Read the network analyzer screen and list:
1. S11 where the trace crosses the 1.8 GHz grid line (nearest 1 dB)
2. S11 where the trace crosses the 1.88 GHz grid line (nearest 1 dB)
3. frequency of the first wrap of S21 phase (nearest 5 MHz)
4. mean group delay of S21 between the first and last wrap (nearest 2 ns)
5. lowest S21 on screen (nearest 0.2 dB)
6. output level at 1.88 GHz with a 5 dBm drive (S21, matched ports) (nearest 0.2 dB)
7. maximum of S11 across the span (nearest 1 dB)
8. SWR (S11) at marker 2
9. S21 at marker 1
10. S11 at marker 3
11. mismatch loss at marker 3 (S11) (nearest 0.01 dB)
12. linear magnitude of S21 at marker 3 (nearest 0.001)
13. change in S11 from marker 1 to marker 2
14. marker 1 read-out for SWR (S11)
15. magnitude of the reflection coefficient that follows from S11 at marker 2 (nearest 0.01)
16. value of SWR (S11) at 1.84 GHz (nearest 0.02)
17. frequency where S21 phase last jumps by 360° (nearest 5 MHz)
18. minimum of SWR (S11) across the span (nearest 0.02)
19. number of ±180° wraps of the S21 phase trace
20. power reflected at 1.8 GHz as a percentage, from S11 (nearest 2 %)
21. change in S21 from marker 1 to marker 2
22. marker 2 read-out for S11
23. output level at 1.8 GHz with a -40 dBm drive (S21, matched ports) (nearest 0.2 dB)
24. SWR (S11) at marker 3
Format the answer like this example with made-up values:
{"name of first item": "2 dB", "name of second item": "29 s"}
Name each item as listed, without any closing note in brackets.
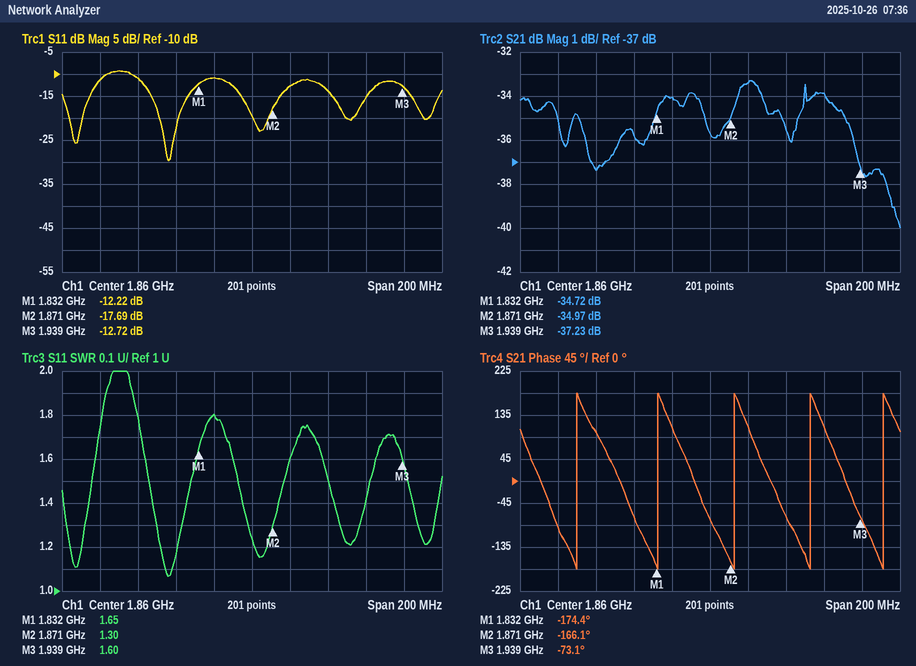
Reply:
{"S11 where the trace crosses the 1.8 GHz grid line": "-11 dB", "S11 where the trace crosses the 1.88 GHz grid line": "-13 dB", "frequency of the first wrap of S21 phase": "1.790 GHz", "mean group delay of S21 between the first and last wrap": "24 ns", "lowest S21 on screen": "-40.0 dB", "output level at 1.88 GHz with a 5 dBm drive (S21, matched ports)": "-28.4 dBm", "maximum of S11 across the span": "-9 dB", "SWR (S11) at marker 2": "1.30", "S21 at marker 1": "-34.72 dB", "S11 at marker 3": "-12.72 dB", "mismatch loss at marker 3 (S11)": "0.24 dB", "linear magnitude of S21 at marker 3": "0.014", "change in S11 from marker 1 to marker 2": "-5.47 dB", "marker 1 read-out for SWR": "1.65", "magnitude of the reflection coefficient that follows from S11 at marker 2": "0.13", "value of SWR (S11) at 1.84 GHz": "1.80", "frequency where S21 phase last jumps by 360°": "1.950 GHz", "minimum of SWR (S11) across the span": "1.06", "number of ±180° wraps of the S21 phase trace": "5", "power reflected at 1.8 GHz as a percentage, from S11": "8 %", "change in S21 from marker 1 to marker 2": "-0.25 dB", "marker 2 read-out for S11": "-17.69 dB", "output level at 1.8 GHz with a -40 dBm drive (S21, matched ports)": "-77.4 dBm", "SWR (S11) at marker 3": "1.60"}
